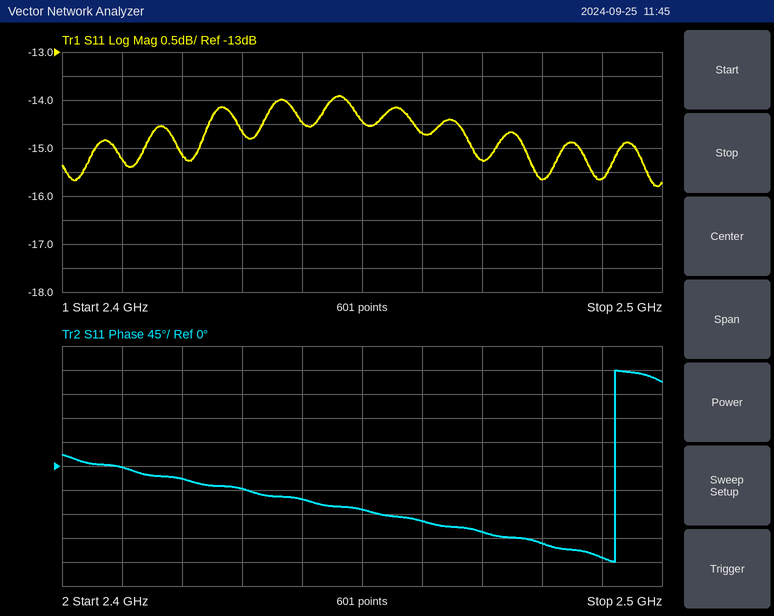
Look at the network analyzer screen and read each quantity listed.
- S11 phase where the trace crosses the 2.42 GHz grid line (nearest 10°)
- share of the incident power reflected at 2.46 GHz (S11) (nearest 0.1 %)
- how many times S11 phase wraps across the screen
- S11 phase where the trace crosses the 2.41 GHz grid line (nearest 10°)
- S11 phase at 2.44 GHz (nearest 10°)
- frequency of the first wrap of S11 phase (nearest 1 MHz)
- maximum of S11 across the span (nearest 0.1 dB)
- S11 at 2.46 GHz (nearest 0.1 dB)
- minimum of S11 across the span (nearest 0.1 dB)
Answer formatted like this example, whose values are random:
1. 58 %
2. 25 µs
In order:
1. -20°
2. 3.4 %
3. 1
4. 0°
5. -60°
6. 2.492 GHz
7. -13.9 dB
8. -14.7 dB
9. -15.8 dB
